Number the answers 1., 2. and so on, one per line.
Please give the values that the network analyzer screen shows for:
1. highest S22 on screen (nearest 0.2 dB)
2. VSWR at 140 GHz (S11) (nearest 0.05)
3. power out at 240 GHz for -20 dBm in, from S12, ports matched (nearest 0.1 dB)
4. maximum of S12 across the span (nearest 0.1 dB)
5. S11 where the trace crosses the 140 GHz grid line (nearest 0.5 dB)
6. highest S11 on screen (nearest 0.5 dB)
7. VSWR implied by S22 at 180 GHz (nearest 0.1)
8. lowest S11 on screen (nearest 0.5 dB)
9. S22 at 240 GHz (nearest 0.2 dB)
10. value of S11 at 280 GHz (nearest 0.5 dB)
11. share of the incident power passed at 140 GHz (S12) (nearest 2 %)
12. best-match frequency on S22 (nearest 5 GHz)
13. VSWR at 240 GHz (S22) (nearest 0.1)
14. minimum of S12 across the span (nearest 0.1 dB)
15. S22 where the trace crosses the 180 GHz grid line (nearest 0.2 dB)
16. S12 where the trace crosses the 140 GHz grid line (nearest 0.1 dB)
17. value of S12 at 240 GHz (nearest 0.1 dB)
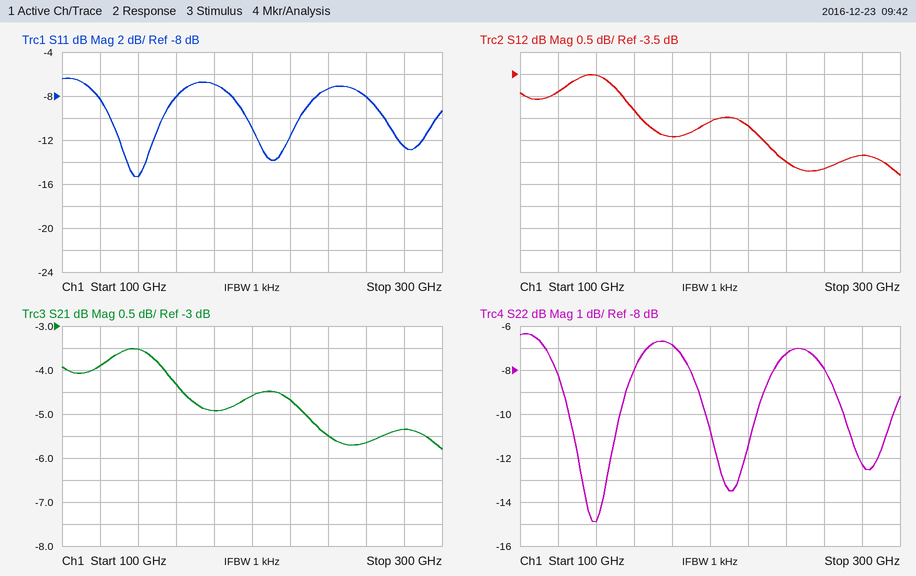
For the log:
1. -6.4 dB
2. 1.40
3. -25.5 dBm
4. -3.5 dB
5. -15.5 dB
6. -6.5 dB
7. 2.7
8. -15.5 dB
9. -7.2 dB
10. -12.5 dB
11. 44 %
12. 140 GHz
13. 2.5
14. -5.8 dB
15. -6.8 dB
16. -3.5 dB
17. -5.5 dB
